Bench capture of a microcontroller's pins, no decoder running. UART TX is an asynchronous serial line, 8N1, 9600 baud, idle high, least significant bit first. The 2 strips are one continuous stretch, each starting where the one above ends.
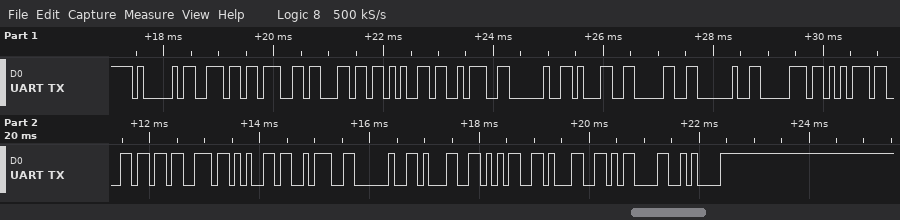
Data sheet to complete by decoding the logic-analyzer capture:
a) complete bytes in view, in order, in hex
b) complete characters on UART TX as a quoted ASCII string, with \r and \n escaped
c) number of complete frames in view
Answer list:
0x41 0x6E 0x67 0x6C 0x65 0x3A 0x20 0x31 0x30 0x20 0x70 0x75 0x6C 0x73 0x65 0x3A 0x20 0x31 0x35 0x31 0x0D 0x0A
"Angle: 10 pulse: 151\r\n"
22
